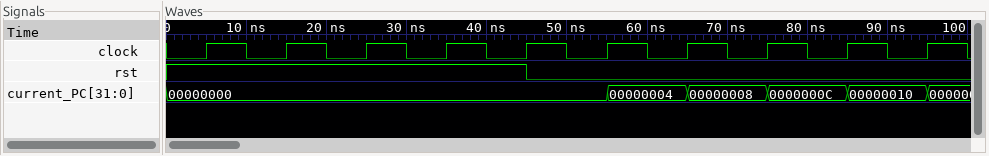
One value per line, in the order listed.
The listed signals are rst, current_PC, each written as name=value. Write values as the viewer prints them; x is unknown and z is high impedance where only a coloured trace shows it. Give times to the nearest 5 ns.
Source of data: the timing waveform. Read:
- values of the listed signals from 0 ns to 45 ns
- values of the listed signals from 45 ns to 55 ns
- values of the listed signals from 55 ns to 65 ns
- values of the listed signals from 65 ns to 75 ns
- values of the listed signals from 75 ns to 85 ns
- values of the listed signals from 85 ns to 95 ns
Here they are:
rst=1, current_PC=00000000
rst=0, current_PC=00000000
rst=0, current_PC=00000004
rst=0, current_PC=00000008
rst=0, current_PC=0000000C
rst=0, current_PC=00000010
